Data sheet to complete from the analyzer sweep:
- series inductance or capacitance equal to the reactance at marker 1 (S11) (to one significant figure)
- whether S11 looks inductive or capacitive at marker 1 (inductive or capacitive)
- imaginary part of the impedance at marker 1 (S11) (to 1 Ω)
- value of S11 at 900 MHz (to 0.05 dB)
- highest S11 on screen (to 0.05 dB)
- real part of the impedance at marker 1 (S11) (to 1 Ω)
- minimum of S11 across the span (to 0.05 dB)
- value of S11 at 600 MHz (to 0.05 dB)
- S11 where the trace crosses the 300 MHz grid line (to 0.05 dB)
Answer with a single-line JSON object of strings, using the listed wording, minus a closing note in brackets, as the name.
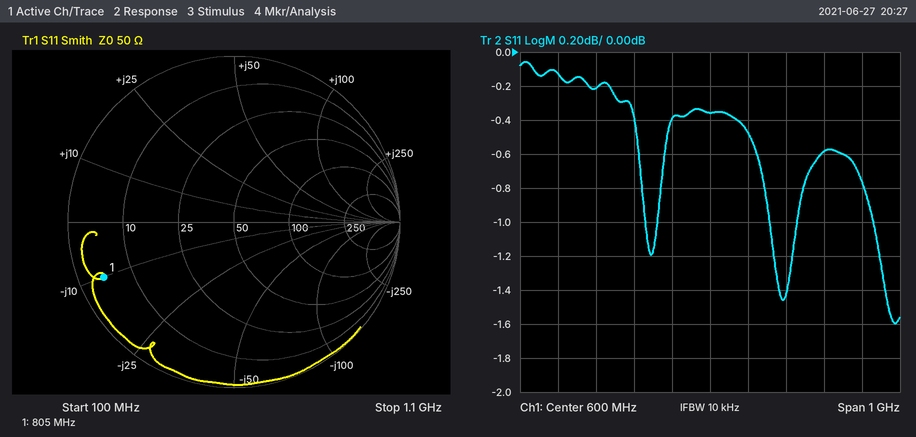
{"series inductance or capacitance equal to the reactance at marker 1 (S11)": "20 pF", "whether S11 looks inductive or capacitive at marker 1": "capacitive", "imaginary part of the impedance at marker 1 (S11)": "-10 Ω", "value of S11 at 900 MHz": "-0.60 dB", "highest S11 on screen": "-0.05 dB", "real part of the impedance at marker 1 (S11)": "4 Ω", "minimum of S11 across the span": "-1.60 dB", "value of S11 at 600 MHz": "-0.35 dB", "S11 where the trace crosses the 300 MHz grid line": "-0.20 dB"}
